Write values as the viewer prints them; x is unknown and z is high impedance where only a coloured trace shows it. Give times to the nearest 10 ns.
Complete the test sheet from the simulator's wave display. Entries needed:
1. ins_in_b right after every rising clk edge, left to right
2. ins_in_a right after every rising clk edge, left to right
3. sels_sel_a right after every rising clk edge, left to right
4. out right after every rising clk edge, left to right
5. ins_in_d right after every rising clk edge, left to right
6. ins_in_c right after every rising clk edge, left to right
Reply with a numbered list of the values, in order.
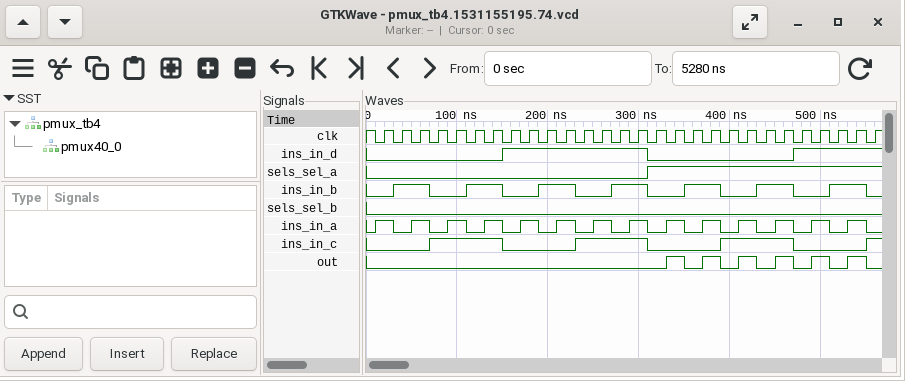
1. 0 1 1 0 0 1 1 0 0 1 1 0 0 1 1 0 0 1 1 0 0 1 1 0 0 1 1 0
2. 1 0 1 0 1 0 1 0 1 0 1 0 1 0 1 0 1 0 1 0 1 0 1 0 1 0 1 0
3. 0 0 0 0 0 0 0 0 0 0 0 0 0 0 0 1 1 1 1 1 1 1 1 1 1 1 1 1
4. 0 0 0 0 0 0 0 0 0 0 0 0 0 0 0 0 1 0 1 0 1 0 1 0 1 0 1 0
5. 0 0 0 0 0 0 0 1 1 1 1 1 1 1 1 0 0 0 0 0 0 0 0 1 1 1 1 1
6. 0 0 0 1 1 1 1 0 0 0 0 1 1 1 1 0 0 0 0 1 1 1 1 0 0 0 0 1
